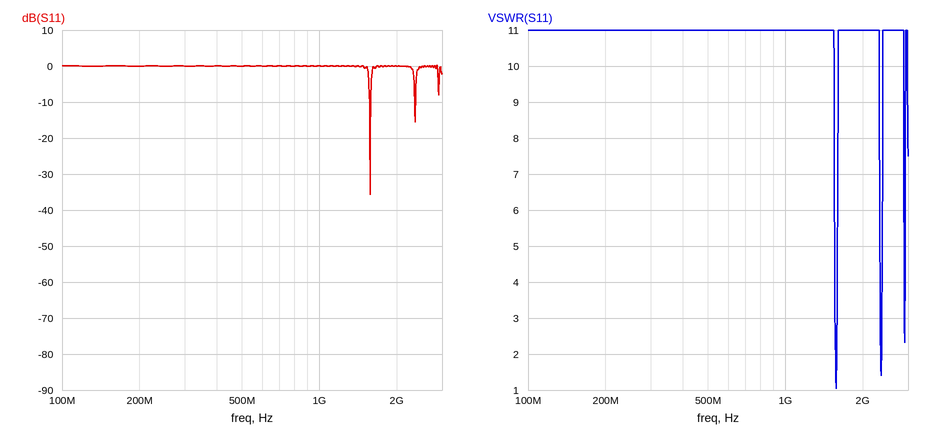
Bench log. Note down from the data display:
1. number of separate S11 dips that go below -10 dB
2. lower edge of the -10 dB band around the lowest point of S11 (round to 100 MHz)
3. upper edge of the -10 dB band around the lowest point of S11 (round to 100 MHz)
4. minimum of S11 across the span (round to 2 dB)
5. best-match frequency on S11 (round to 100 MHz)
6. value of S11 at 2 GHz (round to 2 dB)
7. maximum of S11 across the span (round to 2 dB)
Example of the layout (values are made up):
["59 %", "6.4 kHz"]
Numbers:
["2", "1.6 GHz", "1.6 GHz", "-36 dB", "1.6 GHz", "0 dB", "0 dB"]
